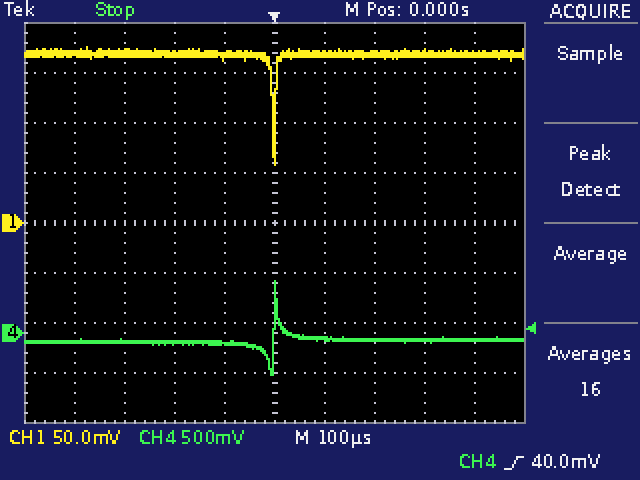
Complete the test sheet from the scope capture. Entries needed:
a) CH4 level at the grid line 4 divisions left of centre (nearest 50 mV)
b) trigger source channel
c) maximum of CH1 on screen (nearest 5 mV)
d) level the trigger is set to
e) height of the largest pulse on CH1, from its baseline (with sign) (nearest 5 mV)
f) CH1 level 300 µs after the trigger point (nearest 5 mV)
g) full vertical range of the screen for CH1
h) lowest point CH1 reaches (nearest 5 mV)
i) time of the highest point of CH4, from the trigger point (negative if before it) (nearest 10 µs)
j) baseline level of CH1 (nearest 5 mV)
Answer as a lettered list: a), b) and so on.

a) -100 mV
b) CH4
c) 175 mV
d) 40.0 mV
e) -110 mV
f) 170 mV
g) 400 mV
h) 60 mV
i) 0 µs
j) 170 mV
